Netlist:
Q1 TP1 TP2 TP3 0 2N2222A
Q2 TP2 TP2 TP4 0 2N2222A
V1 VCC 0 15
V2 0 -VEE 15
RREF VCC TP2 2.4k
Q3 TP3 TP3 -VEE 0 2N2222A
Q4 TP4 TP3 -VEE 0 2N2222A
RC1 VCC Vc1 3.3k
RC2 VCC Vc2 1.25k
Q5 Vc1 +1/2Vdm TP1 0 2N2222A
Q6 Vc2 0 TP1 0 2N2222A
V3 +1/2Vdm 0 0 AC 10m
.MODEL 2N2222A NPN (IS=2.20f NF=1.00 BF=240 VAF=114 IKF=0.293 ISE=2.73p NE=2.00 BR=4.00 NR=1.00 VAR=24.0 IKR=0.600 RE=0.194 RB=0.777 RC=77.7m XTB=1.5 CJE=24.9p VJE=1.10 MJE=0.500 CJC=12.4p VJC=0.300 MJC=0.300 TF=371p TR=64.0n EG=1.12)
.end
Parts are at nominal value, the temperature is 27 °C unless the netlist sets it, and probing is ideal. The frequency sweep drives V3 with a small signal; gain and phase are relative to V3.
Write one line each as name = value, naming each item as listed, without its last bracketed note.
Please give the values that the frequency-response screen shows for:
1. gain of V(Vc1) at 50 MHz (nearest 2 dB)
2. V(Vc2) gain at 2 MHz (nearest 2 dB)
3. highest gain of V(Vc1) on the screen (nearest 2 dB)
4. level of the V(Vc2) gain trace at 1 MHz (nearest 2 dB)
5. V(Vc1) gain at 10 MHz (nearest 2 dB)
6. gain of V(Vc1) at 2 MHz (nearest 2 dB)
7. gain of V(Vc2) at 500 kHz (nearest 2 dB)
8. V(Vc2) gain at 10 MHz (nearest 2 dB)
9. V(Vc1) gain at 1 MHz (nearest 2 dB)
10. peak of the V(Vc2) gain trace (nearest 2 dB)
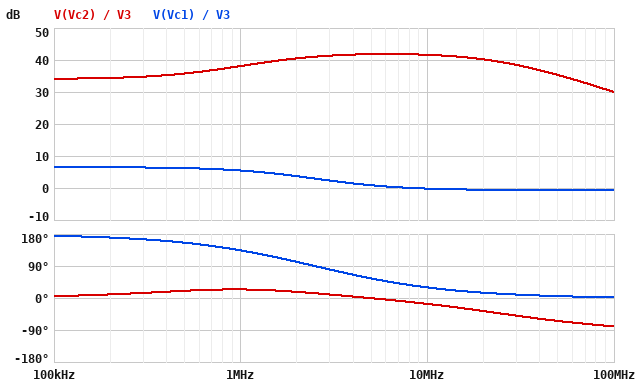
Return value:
gain of V(Vc1) at 50 MHz = 0 dB
V(Vc2) gain at 2 MHz = 40 dB
highest gain of V(Vc1) on the screen = 6 dB
level of the V(Vc2) gain trace at 1 MHz = 38 dB
V(Vc1) gain at 10 MHz = 0 dB
gain of V(Vc1) at 2 MHz = 4 dB
gain of V(Vc2) at 500 kHz = 36 dB
V(Vc2) gain at 10 MHz = 42 dB
V(Vc1) gain at 1 MHz = 6 dB
peak of the V(Vc2) gain trace = 42 dB
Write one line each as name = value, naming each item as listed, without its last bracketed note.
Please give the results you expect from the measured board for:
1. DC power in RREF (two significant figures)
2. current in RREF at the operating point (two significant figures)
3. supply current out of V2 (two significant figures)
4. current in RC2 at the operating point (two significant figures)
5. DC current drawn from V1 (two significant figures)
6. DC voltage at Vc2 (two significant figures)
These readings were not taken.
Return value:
DC power in RREF = 340 mW
current in RREF at the operating point = 12 mA
supply current out of V2 = 24 mA
current in RC2 at the operating point = 6.7 mA
DC current drawn from V1 = 23 mA
DC voltage at Vc2 = 6.6 V
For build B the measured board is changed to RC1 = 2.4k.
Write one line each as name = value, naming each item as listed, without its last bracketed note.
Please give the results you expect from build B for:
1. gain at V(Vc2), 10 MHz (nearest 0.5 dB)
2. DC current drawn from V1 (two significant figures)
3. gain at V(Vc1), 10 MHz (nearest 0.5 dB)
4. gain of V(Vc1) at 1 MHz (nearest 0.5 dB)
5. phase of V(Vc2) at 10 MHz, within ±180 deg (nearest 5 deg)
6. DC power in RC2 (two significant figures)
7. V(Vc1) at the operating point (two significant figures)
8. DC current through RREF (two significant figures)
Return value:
gain at V(Vc2), 10 MHz = 41.0 dB
DC current drawn from V1 = 24 mA
gain at V(Vc1), 10 MHz = 43.5 dB
gain of V(Vc1) at 1 MHz = 47.5 dB
phase of V(Vc2) at 10 MHz, within ±180 deg = -20 deg
DC power in RC2 = 46 mW
V(Vc1) at the operating point = 1.2 V
DC current through RREF = 12 mA
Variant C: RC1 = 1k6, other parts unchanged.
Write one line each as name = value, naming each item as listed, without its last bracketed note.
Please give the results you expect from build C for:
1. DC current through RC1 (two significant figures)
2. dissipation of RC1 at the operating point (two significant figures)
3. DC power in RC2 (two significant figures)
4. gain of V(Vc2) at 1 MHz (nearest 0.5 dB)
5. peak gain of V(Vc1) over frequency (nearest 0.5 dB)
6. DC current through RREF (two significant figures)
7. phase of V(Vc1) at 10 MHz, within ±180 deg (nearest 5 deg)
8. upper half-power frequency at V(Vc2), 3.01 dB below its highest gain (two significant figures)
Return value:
DC current through RC1 = 5.9 mA
dissipation of RC1 at the operating point = 55 mW
DC power in RC2 = 44 mW
gain of V(Vc2) at 1 MHz = 42.0 dB
peak gain of V(Vc1) over frequency = 44.0 dB
DC current through RREF = 12 mA
phase of V(Vc1) at 10 MHz, within ±180 deg = 150 deg
upper half-power frequency at V(Vc2), 3.01 dB below its highest gain = 25 MHz
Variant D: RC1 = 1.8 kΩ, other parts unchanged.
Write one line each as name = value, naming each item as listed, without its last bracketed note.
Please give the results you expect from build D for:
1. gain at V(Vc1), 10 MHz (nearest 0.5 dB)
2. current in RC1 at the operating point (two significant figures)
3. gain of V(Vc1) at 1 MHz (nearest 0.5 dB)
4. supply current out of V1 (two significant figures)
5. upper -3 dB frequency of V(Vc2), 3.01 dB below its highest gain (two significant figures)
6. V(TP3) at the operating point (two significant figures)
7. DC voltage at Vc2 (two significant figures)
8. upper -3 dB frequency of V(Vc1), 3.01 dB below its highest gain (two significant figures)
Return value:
gain at V(Vc1), 10 MHz = 43.5 dB
current in RC1 at the operating point = 5.8 mA
gain of V(Vc1) at 1 MHz = 45.0 dB
supply current out of V1 = 24 mA
upper -3 dB frequency of V(Vc2), 3.01 dB below its highest gain = 25 MHz
V(TP3) at the operating point = -14 V
DC voltage at Vc2 = 7.5 V
upper -3 dB frequency of V(Vc1), 3.01 dB below its highest gain = 15 MHz
